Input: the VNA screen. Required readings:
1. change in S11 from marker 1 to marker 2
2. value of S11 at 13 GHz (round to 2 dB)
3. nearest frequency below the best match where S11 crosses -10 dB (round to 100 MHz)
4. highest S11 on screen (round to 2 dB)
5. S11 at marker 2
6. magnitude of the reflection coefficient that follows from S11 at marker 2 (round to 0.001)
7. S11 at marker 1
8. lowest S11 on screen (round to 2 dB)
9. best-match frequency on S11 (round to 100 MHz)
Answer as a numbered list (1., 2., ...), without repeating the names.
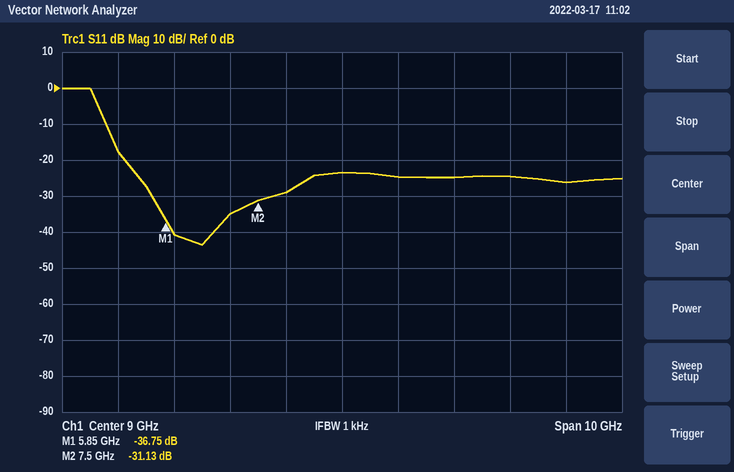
1. 5.62 dB
2. -26 dB
3. 4.8 GHz
4. 0 dB
5. -31.13 dB
6. 0.028
7. -36.75 dB
8. -44 dB
9. 6.5 GHz
